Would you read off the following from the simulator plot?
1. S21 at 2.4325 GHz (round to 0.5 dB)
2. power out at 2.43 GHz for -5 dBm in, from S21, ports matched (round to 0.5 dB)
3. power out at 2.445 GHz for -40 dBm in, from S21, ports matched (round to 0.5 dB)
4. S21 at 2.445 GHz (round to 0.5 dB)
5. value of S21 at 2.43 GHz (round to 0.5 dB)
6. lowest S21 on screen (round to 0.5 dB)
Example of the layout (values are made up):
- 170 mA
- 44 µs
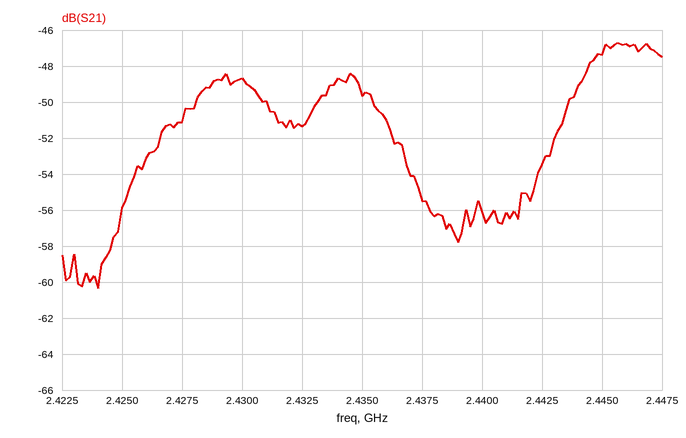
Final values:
- -51.5 dB
- -53.5 dBm
- -87.5 dBm
- -47.5 dB
- -48.5 dB
- -60.5 dB
